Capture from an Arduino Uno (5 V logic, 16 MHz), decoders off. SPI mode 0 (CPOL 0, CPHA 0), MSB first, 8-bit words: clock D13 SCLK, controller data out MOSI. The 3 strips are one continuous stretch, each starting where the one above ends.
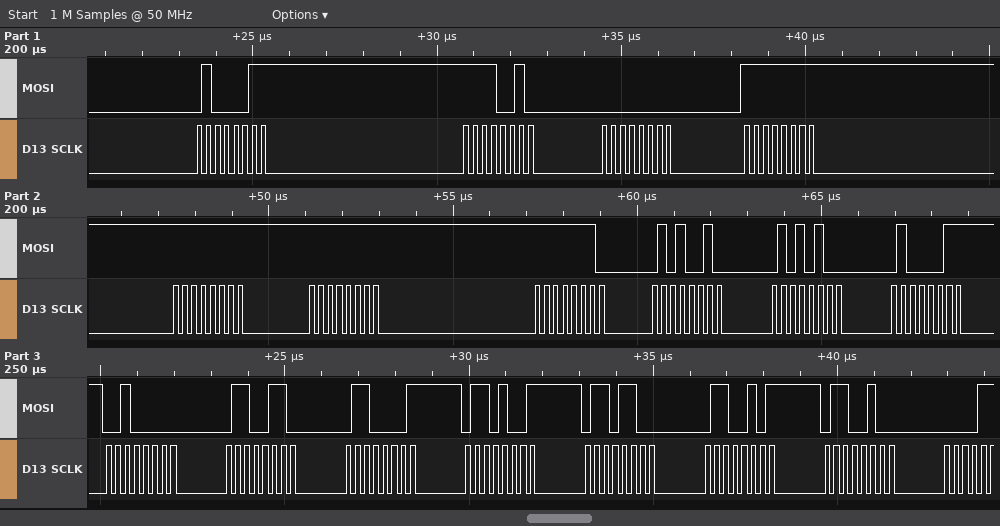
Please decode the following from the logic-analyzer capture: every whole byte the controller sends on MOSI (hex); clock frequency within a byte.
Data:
43 F2 00 FF FF FF FE 52 54 43 20 66 61 69 6C 65 64
4 MHz
